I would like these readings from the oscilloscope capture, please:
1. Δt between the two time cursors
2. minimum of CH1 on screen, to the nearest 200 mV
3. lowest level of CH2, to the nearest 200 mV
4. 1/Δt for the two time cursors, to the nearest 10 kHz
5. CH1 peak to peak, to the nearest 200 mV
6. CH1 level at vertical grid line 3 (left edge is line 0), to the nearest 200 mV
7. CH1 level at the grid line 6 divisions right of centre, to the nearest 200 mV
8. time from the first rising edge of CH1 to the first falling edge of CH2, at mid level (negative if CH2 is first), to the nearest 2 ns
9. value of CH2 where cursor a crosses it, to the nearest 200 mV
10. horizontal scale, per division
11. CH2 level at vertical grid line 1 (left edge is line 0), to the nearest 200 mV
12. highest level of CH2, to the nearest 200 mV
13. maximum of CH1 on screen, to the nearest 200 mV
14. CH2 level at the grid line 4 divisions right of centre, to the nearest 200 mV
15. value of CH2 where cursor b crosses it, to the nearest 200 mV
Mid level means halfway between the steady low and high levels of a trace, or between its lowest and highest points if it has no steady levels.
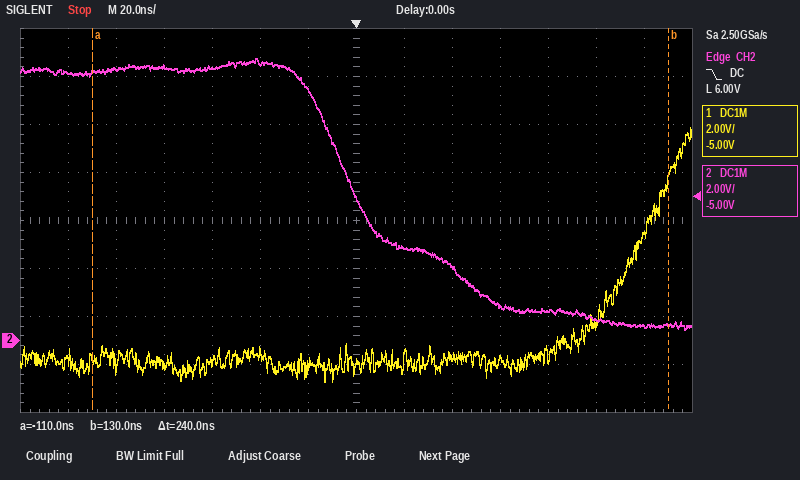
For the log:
240 ns
-1.8 V
400 mV
4.17 MHz
10.6 V
-1.0 V
4.4 V
-116 ns
11.2 V
20 ns
11.2 V
11.8 V
8.8 V
1.2 V
600 mV
